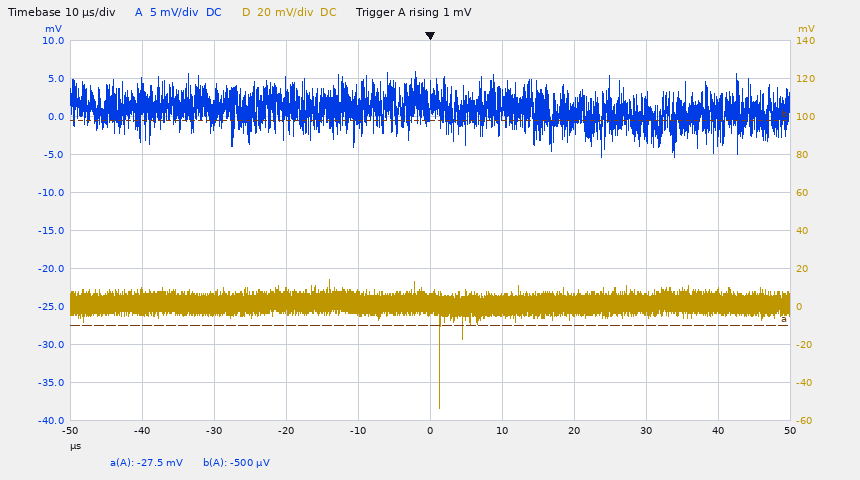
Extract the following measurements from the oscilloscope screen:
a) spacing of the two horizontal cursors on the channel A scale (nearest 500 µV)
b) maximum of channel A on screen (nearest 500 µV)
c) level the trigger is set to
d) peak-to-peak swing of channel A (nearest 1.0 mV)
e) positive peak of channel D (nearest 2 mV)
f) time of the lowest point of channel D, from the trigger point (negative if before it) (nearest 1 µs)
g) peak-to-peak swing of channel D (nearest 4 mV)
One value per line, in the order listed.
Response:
27.0 mV
6.0 mV
1 mV
11.0 mV
14 mV
+1 µs
68 mV
